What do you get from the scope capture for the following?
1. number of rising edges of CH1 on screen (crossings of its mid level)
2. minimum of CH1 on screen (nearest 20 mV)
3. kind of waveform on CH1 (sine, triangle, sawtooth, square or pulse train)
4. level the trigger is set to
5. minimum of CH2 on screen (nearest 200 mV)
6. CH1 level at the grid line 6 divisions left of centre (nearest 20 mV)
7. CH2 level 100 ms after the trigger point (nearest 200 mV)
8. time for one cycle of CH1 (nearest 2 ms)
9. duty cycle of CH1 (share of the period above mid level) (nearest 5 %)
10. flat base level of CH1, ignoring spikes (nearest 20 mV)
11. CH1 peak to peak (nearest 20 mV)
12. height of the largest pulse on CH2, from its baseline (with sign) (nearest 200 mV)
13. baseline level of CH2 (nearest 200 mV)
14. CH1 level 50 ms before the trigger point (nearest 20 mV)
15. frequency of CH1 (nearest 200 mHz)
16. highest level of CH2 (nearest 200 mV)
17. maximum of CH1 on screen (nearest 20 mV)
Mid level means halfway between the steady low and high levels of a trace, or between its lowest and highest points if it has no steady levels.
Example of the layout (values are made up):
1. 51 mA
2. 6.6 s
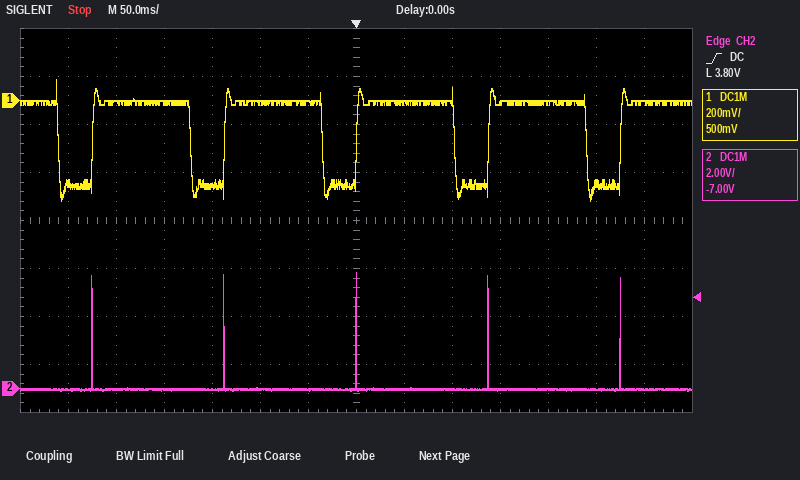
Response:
1. 5
2. -420 mV
3. pulse train
4. 3.80 V
5. 0.0 V
6. -340 mV
7. 0.0 V
8. 138 ms
9. 75 %
10. -360 mV
11. 500 mV
12. +4.8 V
13. 0.0 V
14. 0 mV
15. 7.2 Hz
16. 4.8 V
17. 80 mV
